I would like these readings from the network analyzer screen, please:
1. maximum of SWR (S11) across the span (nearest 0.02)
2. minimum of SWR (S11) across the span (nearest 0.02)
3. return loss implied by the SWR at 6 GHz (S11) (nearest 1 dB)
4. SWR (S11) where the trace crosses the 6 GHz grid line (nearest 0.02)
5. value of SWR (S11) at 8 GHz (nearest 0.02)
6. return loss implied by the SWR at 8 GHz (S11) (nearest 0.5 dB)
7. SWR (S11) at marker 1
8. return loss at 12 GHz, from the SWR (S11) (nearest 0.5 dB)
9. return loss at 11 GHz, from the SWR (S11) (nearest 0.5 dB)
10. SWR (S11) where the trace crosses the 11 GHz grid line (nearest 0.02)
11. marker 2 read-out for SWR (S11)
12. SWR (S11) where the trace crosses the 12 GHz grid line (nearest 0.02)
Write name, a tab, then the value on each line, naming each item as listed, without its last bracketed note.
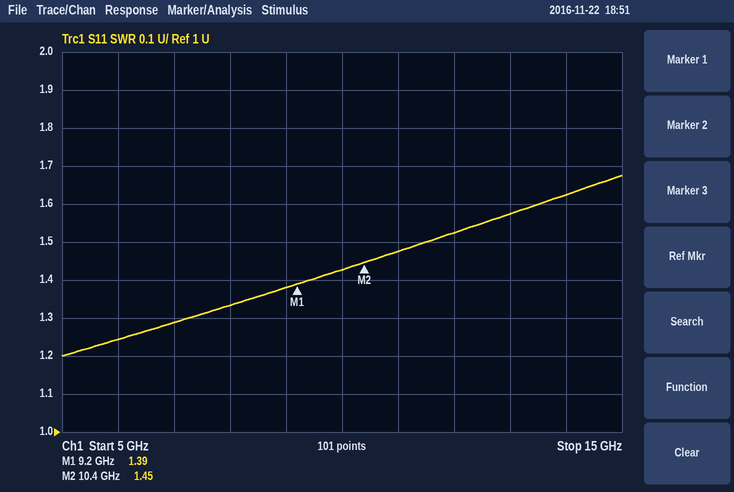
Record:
maximum of SWR (S11) across the span	1.68
minimum of SWR (S11) across the span	1.20
return loss implied by the SWR at 6 GHz (S11)	19 dB
SWR (S11) where the trace crosses the 6 GHz grid line	1.24
value of SWR (S11) at 8 GHz	1.34
return loss implied by the SWR at 8 GHz (S11)	17.0 dB
SWR (S11) at marker 1	1.39
return loss at 12 GHz, from the SWR (S11)	13.5 dB
return loss at 11 GHz, from the SWR (S11)	14.5 dB
SWR (S11) where the trace crosses the 11 GHz grid line	1.48
marker 2 read-out for SWR	1.45
SWR (S11) where the trace crosses the 12 GHz grid line	1.52
